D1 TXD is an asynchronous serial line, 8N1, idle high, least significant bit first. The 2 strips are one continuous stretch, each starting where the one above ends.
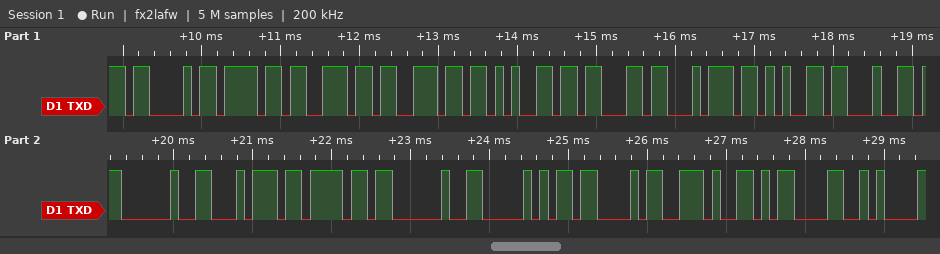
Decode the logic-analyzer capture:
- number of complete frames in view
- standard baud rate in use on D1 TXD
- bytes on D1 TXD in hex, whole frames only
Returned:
18
9600 baud
43 6F 6E 6E 65 63 74 65 64 20 74 6F 20 50 43 2E 0D 0A
